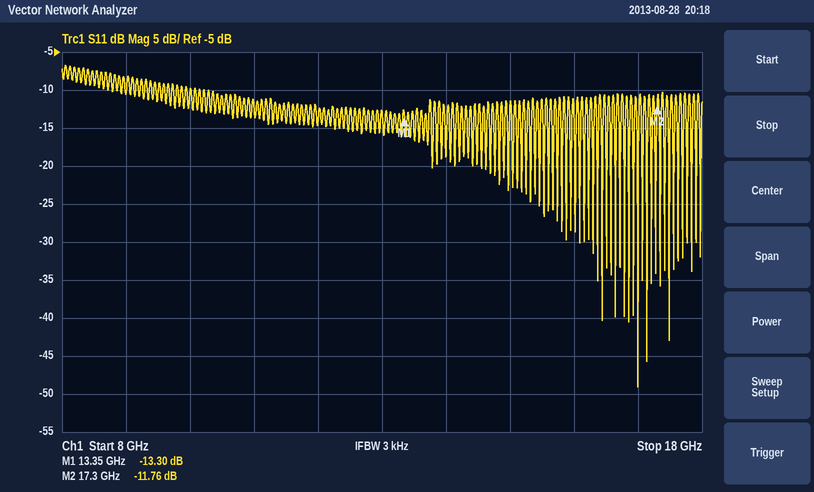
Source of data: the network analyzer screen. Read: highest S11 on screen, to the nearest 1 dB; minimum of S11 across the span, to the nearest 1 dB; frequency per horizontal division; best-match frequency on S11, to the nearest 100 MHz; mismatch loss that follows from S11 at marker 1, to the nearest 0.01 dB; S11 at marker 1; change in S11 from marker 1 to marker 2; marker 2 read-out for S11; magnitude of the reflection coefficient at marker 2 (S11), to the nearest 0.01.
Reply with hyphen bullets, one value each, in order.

- -7 dB
- -49 dB
- 1 GHz
- 17.0 GHz
- 0.21 dB
- -13.30 dB
- 1.54 dB
- -11.76 dB
- 0.26
